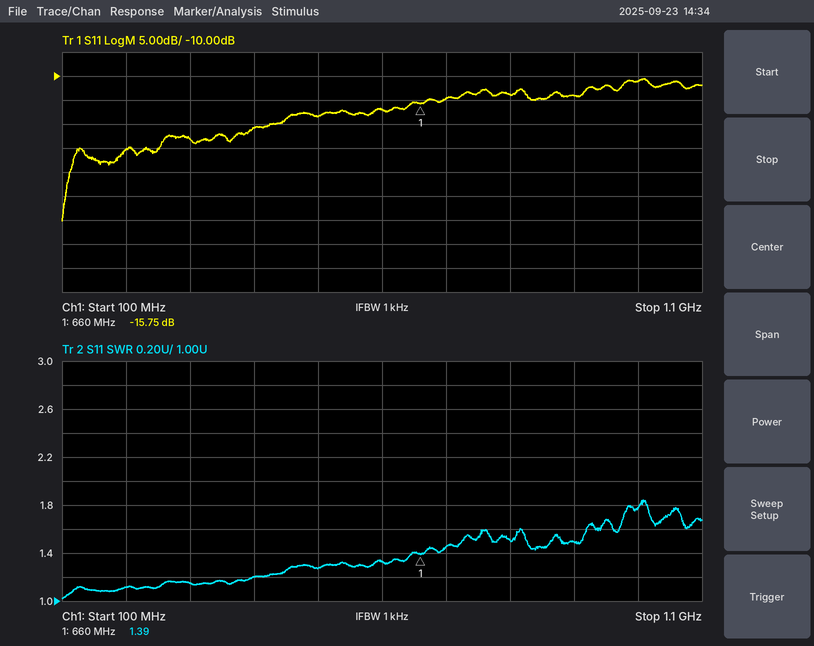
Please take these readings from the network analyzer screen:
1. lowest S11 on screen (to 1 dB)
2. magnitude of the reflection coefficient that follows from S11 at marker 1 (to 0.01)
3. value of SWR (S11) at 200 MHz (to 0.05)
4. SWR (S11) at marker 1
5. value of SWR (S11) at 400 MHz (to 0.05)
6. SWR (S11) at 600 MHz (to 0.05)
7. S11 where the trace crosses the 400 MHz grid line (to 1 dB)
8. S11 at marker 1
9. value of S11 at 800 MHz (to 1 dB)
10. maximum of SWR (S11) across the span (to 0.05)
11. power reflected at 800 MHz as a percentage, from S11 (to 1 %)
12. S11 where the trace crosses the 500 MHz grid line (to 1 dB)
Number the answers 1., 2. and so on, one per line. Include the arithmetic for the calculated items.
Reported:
1. -40 dB
2. 10^(-15.75/20) ≈ 0.16
3. 1.10
4. 1.39
5. 1.20
6. 1.35
7. -21 dB
8. -15.75 dB
9. -14 dB
10. 1.85
11. 10^(-14/10) ≈ 4 %
12. -18 dB
